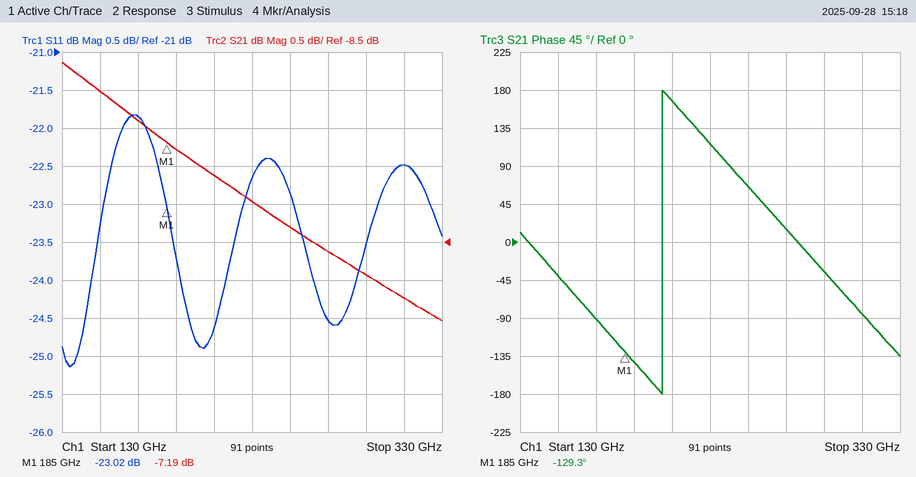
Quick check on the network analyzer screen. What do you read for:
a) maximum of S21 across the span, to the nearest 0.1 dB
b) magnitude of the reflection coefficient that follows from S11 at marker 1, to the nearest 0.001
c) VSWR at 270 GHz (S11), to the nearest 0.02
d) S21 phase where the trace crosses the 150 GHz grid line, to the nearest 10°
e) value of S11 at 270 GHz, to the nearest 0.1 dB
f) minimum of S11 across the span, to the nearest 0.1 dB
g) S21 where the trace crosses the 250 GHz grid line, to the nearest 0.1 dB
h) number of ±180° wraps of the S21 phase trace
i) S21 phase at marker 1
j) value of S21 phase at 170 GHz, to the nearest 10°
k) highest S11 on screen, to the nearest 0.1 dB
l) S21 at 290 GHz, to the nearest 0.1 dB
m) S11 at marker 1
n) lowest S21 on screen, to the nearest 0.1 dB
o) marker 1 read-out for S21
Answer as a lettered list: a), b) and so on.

a) -6.1 dB
b) 0.071
c) 1.12
d) -40°
e) -24.5 dB
f) -25.1 dB
g) -8.3 dB
h) 1
i) -129.3°
j) -90°
k) -21.8 dB
l) -8.9 dB
m) -23.02 dB
n) -9.5 dB
o) -7.19 dB
